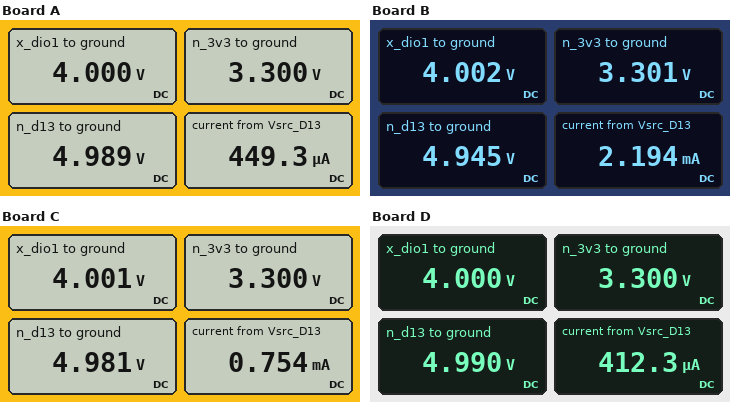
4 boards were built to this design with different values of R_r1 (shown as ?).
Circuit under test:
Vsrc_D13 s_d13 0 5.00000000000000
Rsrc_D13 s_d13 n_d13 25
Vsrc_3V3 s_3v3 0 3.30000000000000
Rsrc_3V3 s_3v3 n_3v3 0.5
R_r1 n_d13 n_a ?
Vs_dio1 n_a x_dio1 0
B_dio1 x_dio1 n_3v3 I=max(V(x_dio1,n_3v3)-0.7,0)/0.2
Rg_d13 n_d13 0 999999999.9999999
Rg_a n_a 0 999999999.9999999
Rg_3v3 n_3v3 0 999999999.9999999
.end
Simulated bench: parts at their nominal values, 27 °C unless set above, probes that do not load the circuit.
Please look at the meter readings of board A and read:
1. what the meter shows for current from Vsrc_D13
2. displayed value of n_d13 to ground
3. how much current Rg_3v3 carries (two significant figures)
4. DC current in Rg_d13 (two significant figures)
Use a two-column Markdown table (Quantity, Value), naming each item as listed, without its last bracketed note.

| Quantity | Value |
|---|---|
| what the meter shows for current from Vsrc_D13 | 449.3 µA |
| displayed value of n_d13 to ground | 4.989 V |
| how much current Rg_3v3 carries | 3.3 nA |
| DC current in Rg_d13 | 5.0 nA |
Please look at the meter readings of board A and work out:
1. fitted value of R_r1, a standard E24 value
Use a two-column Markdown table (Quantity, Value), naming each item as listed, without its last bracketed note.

| Quantity | Value |
|---|---|
| fitted value of R_r1, a standard E24 value | 2.2 kΩ |
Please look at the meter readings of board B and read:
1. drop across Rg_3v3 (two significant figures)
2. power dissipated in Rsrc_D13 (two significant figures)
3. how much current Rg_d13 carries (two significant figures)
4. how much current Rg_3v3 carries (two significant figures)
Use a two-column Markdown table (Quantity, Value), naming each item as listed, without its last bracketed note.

| Quantity | Value |
|---|---|
| drop across Rg_3v3 | 3.3 V |
| power dissipated in Rsrc_D13 | 120 µW |
| how much current Rg_d13 carries | 4.9 nA |
| how much current Rg_3v3 carries | 3.3 nA |
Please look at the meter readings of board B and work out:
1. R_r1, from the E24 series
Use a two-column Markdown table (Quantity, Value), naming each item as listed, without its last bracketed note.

| Quantity | Value |
|---|---|
| R_r1, from the E24 series | 430 Ω |
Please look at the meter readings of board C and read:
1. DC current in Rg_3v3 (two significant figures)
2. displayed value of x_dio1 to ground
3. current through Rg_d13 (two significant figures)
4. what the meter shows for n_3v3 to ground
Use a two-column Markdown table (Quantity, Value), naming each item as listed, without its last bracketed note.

| Quantity | Value |
|---|---|
| DC current in Rg_3v3 | 3.3 nA |
| displayed value of x_dio1 to ground | 4.001 V |
| current through Rg_d13 | 5.0 nA |
| what the meter shows for n_3v3 to ground | 3.300 V |
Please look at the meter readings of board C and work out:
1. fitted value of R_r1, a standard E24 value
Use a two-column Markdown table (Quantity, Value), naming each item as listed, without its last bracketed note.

| Quantity | Value |
|---|---|
| fitted value of R_r1, a standard E24 value | 1.3 kΩ |
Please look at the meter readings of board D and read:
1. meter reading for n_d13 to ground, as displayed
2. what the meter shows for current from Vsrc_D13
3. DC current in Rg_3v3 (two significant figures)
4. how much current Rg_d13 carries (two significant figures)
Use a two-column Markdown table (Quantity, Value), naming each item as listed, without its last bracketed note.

| Quantity | Value |
|---|---|
| meter reading for n_d13 to ground, as displayed | 4.990 V |
| what the meter shows for current from Vsrc_D13 | 412.3 µA |
| DC current in Rg_3v3 | 3.3 nA |
| how much current Rg_d13 carries | 5.0 nA |
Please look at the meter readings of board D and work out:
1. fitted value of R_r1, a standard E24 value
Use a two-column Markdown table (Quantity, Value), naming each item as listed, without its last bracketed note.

| Quantity | Value |
|---|---|
| fitted value of R_r1, a standard E24 value | 2.4 kΩ |
